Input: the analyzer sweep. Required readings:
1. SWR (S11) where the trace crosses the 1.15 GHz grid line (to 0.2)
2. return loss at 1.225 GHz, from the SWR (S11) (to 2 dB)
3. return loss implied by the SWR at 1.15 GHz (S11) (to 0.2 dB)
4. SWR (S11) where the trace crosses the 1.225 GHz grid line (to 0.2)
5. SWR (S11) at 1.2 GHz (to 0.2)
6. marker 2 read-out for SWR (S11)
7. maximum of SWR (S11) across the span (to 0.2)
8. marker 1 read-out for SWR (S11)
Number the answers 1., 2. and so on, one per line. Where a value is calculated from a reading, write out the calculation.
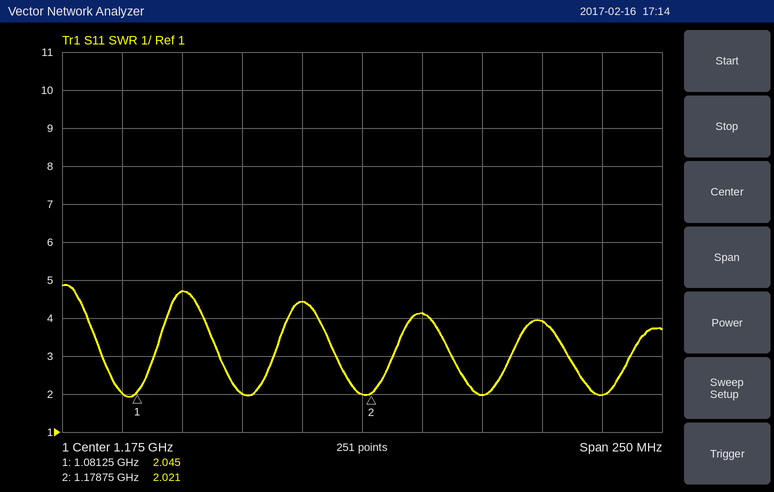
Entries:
1. 4.4
2. −20 log10((2 − 1)/(2 + 1)) ≈ 10 dB
3. −20 log10((4.4 − 1)/(4.4 + 1)) ≈ 4.0 dB
4. 2.0
5. 4.2
6. 2.021
7. 4.8
8. 2.045
